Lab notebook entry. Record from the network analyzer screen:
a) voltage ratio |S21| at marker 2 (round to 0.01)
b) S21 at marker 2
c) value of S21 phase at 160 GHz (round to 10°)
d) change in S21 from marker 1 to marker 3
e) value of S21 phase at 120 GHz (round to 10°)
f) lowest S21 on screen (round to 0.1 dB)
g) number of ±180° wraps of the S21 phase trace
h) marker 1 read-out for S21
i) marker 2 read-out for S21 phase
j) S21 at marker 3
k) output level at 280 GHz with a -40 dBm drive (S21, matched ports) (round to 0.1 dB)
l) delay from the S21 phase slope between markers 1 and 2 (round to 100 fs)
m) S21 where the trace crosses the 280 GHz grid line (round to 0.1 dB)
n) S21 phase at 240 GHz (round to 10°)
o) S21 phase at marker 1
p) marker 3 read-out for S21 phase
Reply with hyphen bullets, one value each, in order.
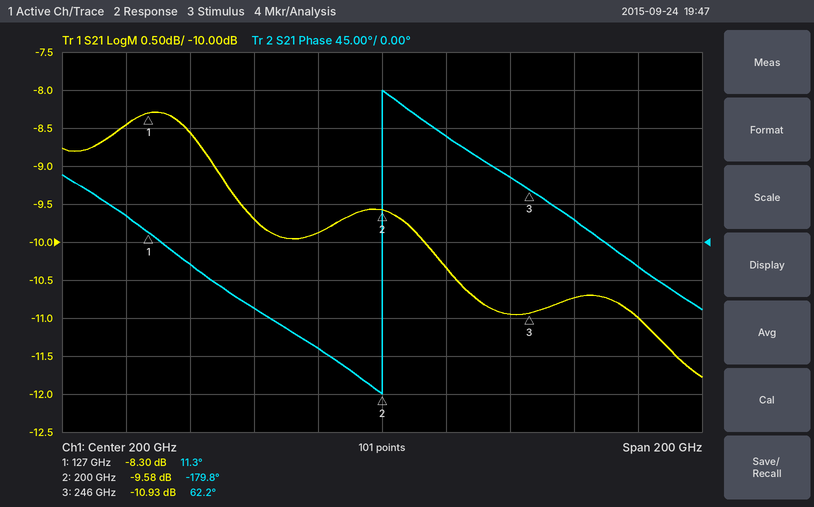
- 0.33
- -9.58 dB
- -80°
- -2.63 dB
- 30°
- -11.8 dB
- 1
- -8.30 dB
- -179.8°
- -10.93 dB
- -51.0 dBm
- 7.3 ps
- -11.0 dB
- 80°
- 11.3°
- 62.2°
